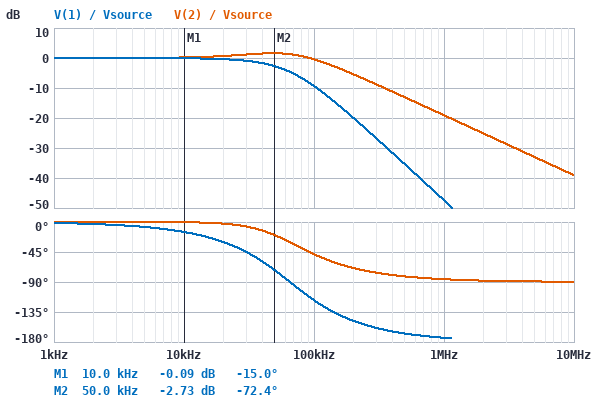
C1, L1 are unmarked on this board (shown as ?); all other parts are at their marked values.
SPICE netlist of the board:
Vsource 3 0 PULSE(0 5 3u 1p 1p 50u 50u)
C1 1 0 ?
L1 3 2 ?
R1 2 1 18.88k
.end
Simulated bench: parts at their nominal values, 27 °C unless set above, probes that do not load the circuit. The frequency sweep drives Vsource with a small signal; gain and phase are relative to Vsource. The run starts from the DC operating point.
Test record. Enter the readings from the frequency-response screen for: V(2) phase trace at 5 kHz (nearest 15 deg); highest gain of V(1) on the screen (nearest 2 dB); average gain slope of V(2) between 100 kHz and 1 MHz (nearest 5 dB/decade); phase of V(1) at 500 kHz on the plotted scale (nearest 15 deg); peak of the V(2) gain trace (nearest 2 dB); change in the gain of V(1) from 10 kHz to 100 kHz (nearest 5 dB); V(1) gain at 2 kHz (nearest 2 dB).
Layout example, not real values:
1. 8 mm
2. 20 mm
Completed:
1. 0 deg
2. 0 dB
3. -20 dB/decade
4. -165 deg
5. 2 dB
6. -10 dB
7. 0 dB
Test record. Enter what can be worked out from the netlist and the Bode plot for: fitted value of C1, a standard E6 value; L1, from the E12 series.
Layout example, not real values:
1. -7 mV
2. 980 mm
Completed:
1. 220 pF
2. 27 mH
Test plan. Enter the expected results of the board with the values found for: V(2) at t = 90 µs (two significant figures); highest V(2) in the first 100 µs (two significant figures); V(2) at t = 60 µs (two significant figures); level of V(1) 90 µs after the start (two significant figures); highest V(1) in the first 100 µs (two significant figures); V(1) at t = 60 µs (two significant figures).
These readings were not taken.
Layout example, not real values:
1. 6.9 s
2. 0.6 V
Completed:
1. 5.0 V
2. 5.8 V
3. 5.0 V
4. 5.0 V
5. 5.0 V
6. 5.0 V
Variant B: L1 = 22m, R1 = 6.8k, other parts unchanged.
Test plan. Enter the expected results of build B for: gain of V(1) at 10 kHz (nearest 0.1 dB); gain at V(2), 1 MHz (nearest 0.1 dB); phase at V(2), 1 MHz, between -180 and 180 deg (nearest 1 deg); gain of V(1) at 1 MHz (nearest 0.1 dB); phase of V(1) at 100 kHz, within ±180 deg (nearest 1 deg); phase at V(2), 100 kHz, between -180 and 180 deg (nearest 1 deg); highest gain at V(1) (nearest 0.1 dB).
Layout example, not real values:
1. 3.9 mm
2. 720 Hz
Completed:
1. 0.1 dB
2. -26.1 dB
3. -93 deg
4. -45.6 dB
5. -134 deg
6. -91 deg
7. 3.9 dB
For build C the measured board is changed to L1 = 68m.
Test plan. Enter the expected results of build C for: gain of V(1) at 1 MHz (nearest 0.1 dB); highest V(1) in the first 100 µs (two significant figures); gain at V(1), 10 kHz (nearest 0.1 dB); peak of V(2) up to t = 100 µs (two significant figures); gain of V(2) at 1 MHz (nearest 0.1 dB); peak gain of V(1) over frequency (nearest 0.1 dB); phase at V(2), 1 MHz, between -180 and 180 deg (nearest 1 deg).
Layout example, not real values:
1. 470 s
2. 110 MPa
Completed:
1. -55.4 dB
2. 5.7 V
3. 0.2 dB
4. 6.4 V
5. -27.1 dB
6. 0.9 dB
7. -90 deg
